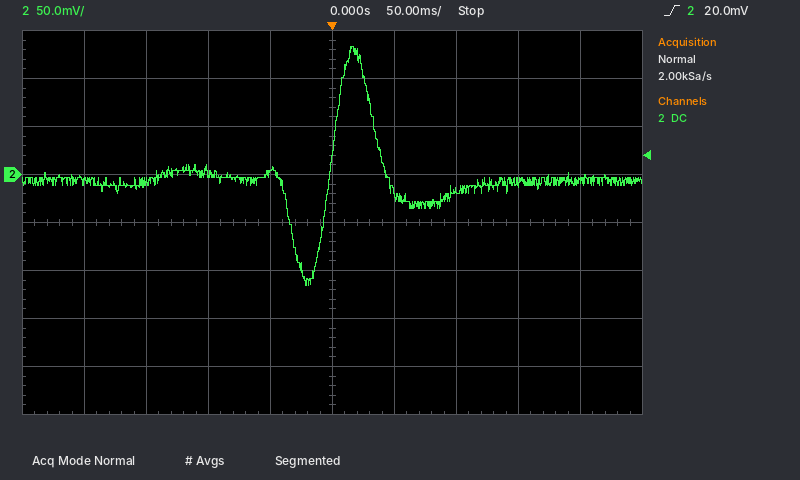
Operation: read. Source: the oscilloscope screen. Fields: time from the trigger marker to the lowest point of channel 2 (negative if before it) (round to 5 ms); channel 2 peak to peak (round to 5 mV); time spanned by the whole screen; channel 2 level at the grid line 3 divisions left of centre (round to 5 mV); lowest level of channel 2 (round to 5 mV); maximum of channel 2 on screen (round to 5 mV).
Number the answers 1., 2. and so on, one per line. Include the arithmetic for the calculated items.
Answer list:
1. -20 ms
2. 135 mV − (-115 mV) = 250 mV
3. 500 ms
4. -10 mV
5. -115 mV
6. 135 mV
